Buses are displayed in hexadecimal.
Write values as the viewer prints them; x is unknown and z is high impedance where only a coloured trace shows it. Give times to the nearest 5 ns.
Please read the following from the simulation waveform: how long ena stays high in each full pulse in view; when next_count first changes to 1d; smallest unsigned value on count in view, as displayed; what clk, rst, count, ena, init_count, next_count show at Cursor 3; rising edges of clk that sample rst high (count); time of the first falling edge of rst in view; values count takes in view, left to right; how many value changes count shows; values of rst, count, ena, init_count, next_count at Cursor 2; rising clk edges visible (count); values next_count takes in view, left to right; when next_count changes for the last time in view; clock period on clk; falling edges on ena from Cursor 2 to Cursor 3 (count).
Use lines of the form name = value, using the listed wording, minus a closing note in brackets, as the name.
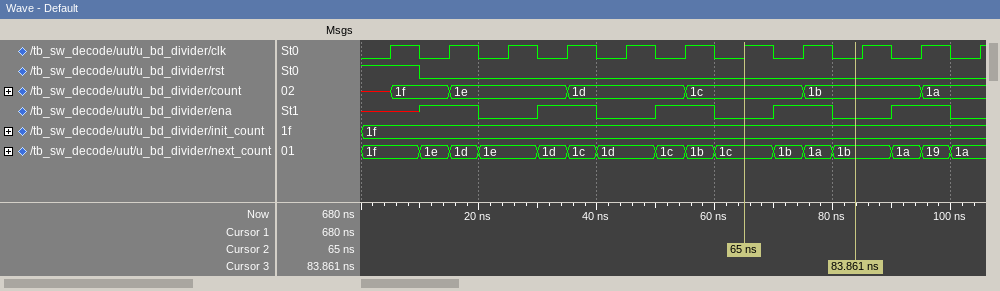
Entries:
how long ena stays high in each full pulse in view = 10 ns, 10 ns, 10 ns, 10 ns
when next_count first changes to 1d = 15 ns
smallest unsigned value on count in view, as displayed = 1a
what clk, rst, count, ena, init_count, next_count show at Cursor 3 = clk=0, rst=0, count=1b, ena=0, init_count=1f, next_count=1b
rising edges of clk that sample rst high = 1
time of the first falling edge of rst in view = 10 ns
values count takes in view, left to right = x, 1f, 1e, 1d, 1c, 1b, 1a
how many value changes count shows = 6
values of rst, count, ena, init_count, next_count at Cursor 2 = rst=0, count=1c, ena=0, init_count=1f, next_count=1c
rising clk edges visible = 11
values next_count takes in view, left to right = 1f, 1e, 1d, 1e, 1d, 1c, 1d, 1c, 1b, 1c, 1b, 1a, 1b, 1a, 19, 1a
when next_count changes for the last time in view = 100 ns
clock period on clk = 10 ns
falling edges on ena from Cursor 2 to Cursor 3 = 1
